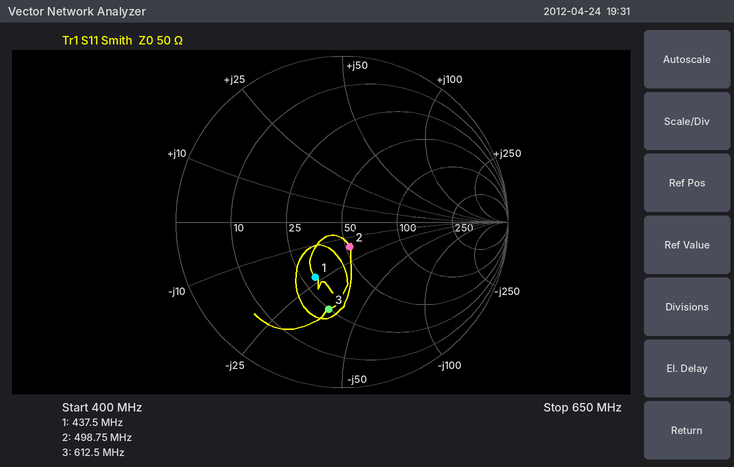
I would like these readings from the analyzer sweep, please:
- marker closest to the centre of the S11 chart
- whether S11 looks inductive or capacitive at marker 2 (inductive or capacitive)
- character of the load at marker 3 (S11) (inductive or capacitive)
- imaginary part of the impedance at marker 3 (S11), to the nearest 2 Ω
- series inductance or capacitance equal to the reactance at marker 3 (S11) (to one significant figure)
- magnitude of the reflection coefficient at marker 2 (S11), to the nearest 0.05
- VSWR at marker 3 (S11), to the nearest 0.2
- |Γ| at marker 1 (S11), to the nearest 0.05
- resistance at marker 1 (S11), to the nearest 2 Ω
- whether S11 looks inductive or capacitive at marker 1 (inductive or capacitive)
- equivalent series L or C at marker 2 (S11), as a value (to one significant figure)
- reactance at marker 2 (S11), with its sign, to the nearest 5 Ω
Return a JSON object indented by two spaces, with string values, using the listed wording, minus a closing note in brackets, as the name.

{
  "marker closest to the centre of the S11 chart": "marker 2",
  "whether S11 looks inductive or capacitive at marker 2": "capacitive",
  "character of the load at marker 3 (S11)": "capacitive",
  "imaginary part of the impedance at marker 3 (S11), to the nearest 2 Ω": "-36 Ω",
  "series inductance or capacitance equal to the reactance at marker 3 (S11)": "7 pF",
  "magnitude of the reflection coefficient at marker 2 (S11), to the nearest 0.05": "0.15",
  "VSWR at marker 3 (S11), to the nearest 0.2": "3.2",
  "|Γ| at marker 1 (S11), to the nearest 0.05": "0.35",
  "resistance at marker 1 (S11), to the nearest 2 Ω": "30 Ω",
  "whether S11 looks inductive or capacitive at marker 1": "capacitive",
  "equivalent series L or C at marker 2 (S11), as a value": "20 pF",
  "reactance at marker 2 (S11), with its sign, to the nearest 5 Ω": "-15 Ω"
}
